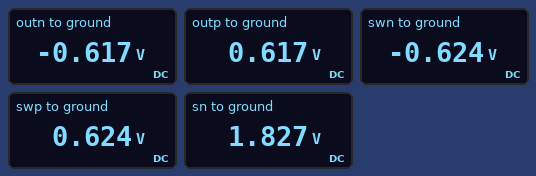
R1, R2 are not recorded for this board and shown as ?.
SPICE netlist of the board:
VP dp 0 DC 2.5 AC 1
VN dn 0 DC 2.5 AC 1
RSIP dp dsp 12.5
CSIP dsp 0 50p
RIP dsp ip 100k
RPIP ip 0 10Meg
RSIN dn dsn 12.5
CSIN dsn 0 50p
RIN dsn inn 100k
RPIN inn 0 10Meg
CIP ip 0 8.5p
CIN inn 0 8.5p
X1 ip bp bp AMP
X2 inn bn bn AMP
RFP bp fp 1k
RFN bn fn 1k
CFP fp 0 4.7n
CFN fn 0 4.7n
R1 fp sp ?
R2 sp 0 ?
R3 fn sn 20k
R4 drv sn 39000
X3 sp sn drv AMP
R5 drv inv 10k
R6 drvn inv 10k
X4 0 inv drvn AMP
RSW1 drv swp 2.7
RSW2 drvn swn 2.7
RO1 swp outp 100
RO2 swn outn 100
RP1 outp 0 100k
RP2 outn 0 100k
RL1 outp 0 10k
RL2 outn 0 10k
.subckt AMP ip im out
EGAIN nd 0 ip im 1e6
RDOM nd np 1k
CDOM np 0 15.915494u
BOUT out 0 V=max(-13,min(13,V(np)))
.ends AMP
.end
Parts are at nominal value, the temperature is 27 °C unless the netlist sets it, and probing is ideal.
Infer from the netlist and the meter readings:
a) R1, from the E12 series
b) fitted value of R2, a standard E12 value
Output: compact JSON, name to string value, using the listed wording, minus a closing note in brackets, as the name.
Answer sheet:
{"R1, from the E12 series": "6.8 kΩ", "fitted value of R2, a standard E12 value": "22 kΩ"}
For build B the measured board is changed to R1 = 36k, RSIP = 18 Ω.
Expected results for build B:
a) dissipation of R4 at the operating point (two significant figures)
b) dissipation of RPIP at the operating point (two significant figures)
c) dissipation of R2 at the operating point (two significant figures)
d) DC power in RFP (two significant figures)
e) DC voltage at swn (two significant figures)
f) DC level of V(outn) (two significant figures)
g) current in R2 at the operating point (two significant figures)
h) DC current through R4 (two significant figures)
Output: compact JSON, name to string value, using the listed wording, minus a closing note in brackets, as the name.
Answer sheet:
{"dissipation of R4 at the operating point": "210 µW", "dissipation of RPIP at the operating point": "610 nW", "dissipation of R2 at the operating point": "39 µW", "DC power in RFP": "1.8 µW", "DC voltage at swn": "2.0 V", "DC level of V(outn)": "1.9 V", "current in R2 at the operating point": "42 µA", "DC current through R4": "74 µA"}
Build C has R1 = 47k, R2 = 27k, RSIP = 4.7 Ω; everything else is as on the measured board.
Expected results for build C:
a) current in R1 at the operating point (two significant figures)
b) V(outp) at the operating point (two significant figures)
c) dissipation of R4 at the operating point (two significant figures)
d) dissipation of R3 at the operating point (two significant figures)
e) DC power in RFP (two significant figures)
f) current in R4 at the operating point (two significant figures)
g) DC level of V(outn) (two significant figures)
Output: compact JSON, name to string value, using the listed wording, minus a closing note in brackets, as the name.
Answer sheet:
{"current in R1 at the operating point": "33 µA", "V(outp) at the operating point": "-2.0 V", "dissipation of R4 at the operating point": "220 µW", "dissipation of R3 at the operating point": "110 µW", "DC power in RFP": "1.1 µW", "current in R4 at the operating point": "75 µA", "DC level of V(outn)": "2.0 V"}
